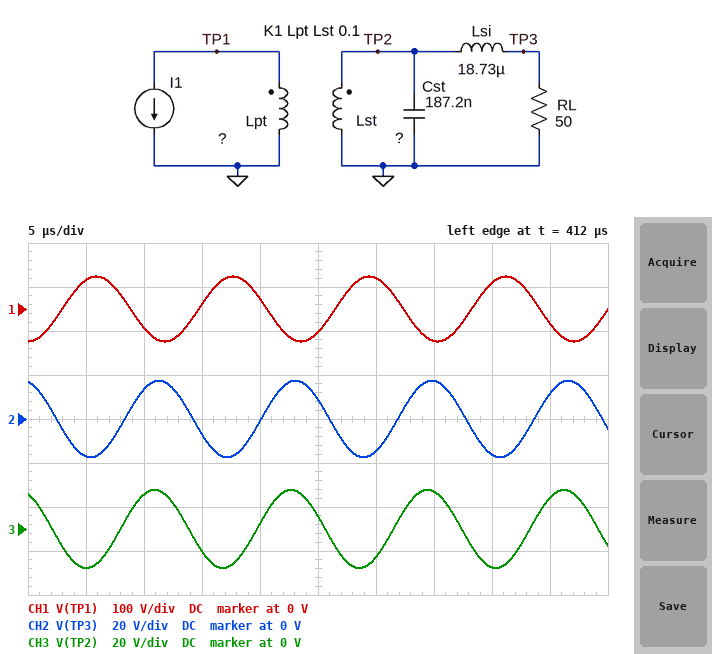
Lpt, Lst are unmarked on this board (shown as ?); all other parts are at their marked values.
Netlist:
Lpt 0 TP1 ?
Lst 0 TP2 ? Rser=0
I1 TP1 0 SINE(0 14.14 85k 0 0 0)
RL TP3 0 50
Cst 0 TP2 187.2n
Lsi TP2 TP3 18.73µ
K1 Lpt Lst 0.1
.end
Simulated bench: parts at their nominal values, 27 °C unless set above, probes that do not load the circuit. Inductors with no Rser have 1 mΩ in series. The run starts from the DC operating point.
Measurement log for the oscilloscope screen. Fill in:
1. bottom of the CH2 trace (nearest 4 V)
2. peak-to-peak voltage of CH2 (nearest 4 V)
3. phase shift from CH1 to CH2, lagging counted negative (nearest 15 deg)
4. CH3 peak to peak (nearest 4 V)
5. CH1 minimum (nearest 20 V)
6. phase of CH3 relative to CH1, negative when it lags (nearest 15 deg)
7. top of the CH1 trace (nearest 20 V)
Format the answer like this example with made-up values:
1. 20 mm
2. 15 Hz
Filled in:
1. -16 V
2. 36 V
3. -165 deg
4. 36 V
5. -80 V
6. -150 deg
7. 80 V
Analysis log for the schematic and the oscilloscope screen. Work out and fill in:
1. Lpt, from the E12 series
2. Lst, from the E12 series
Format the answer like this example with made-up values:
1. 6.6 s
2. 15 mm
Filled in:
1. 10 µH
2. 33 µH
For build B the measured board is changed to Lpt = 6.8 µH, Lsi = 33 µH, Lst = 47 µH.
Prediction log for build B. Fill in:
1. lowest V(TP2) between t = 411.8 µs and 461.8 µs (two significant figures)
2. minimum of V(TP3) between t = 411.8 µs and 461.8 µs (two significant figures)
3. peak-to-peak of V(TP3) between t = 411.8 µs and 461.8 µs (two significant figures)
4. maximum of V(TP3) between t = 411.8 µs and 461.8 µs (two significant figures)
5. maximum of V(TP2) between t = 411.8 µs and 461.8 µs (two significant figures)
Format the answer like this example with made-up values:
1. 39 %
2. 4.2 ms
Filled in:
1. -9.5 V
2. -8.9 V
3. 18 V
4. 8.9 V
5. 9.5 V
